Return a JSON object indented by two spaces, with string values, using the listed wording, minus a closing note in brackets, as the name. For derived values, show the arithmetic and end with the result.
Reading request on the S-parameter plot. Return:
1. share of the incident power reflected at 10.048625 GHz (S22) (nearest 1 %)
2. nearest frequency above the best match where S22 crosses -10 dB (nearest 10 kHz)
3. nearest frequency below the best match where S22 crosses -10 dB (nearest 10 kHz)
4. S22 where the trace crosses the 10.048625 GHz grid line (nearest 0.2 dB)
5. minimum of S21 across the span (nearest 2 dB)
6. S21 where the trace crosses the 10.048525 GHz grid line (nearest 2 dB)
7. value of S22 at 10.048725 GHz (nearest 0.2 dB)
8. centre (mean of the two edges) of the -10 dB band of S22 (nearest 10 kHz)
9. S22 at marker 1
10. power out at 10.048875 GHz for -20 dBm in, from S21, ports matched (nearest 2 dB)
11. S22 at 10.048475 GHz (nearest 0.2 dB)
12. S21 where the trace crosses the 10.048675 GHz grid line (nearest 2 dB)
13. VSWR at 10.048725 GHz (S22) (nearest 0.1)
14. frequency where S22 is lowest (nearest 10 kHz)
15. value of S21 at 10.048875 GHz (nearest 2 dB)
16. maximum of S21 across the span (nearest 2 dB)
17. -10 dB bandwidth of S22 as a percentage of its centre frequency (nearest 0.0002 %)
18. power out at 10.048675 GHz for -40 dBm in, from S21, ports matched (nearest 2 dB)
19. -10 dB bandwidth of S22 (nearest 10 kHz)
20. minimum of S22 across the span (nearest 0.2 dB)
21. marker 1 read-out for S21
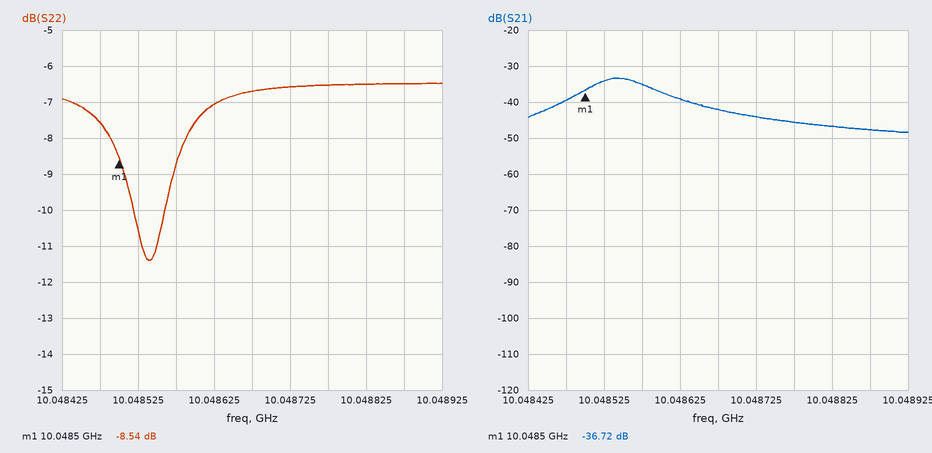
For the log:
{
  "share of the incident power reflected at 10.048625 GHz (S22)": "10^(-7/10) ≈ 20 %",
  "nearest frequency above the best match where S22 crosses -10 dB": "10.04856 GHz",
  "nearest frequency below the best match where S22 crosses -10 dB": "10.04852 GHz",
  "S22 where the trace crosses the 10.048625 GHz grid line": "-7.0 dB",
  "minimum of S21 across the span": "-48 dB",
  "S21 where the trace crosses the 10.048525 GHz grid line": "-34 dB",
  "value of S22 at 10.048725 GHz": "-6.6 dB",
  "centre (mean of the two edges) of the -10 dB band of S22": "10.04854 GHz",
  "S22 at marker 1": "-8.54 dB",
  "power out at 10.048875 GHz for -20 dBm in, from S21, ports matched": "-20 dBm + (-48 dB) = -68 dBm",
  "S22 at 10.048475 GHz": "-7.6 dB",
  "S21 where the trace crosses the 10.048675 GHz grid line": "-42 dB",
  "VSWR at 10.048725 GHz (S22)": "|Γ| = 10^(-6.6/20) = 0.4677; VSWR = (1 + 0.4677)/(1 − 0.4677) ≈ 2.8",
  "frequency where S22 is lowest": "10.04854 GHz",
  "value of S21 at 10.048875 GHz": "-48 dB",
  "maximum of S21 across the span": "-34 dB",
  "-10 dB bandwidth of S22 as a percentage of its centre frequency": "40 kHz / 10.0485 GHz ≈ 0.0004 %",
  "power out at 10.048675 GHz for -40 dBm in, from S21, ports matched": "-40 dBm + (-42 dB) = -82 dBm",
  "-10 dB bandwidth of S22": "10.04856 GHz − 10.04852 GHz = 40 kHz",
  "minimum of S22 across the span": "-11.4 dB",
  "marker 1 read-out for S21": "-36.72 dB"
}
